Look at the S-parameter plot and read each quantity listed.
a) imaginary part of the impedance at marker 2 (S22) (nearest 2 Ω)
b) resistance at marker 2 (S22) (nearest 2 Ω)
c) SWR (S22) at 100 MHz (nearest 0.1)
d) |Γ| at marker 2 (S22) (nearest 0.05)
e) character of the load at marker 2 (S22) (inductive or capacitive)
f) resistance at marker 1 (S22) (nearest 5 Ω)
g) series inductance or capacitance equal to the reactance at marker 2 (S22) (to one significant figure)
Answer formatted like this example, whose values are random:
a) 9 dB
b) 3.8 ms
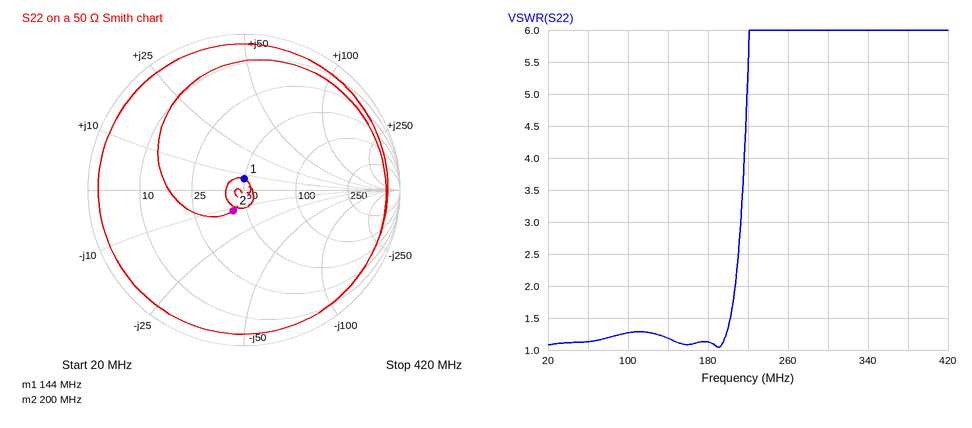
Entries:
a) -12 Ω
b) 42 Ω
c) 1.3
d) 0.15
e) capacitive
f) 50 Ω
g) 70 pF
